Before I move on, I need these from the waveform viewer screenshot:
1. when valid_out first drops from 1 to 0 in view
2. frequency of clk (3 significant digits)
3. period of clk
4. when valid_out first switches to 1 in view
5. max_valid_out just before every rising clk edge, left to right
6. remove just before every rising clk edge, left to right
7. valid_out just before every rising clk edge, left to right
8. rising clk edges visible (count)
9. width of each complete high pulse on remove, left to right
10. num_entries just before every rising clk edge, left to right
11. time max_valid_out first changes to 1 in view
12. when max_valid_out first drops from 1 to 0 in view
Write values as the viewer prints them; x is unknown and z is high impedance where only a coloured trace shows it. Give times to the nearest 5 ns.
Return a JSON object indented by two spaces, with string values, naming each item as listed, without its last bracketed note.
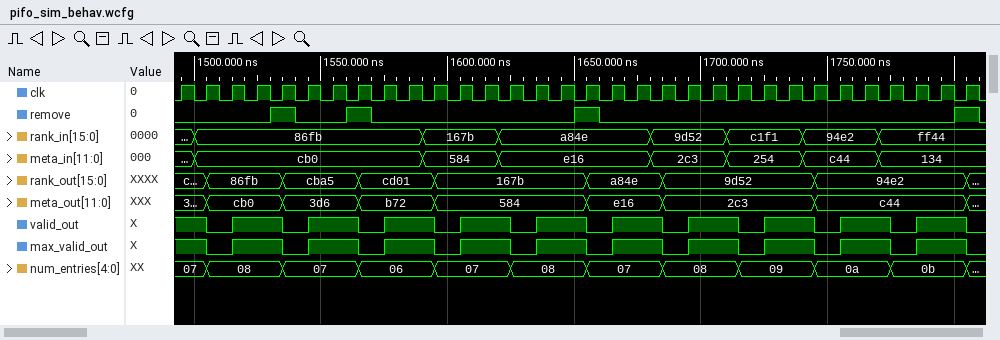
{
  "when valid_out first drops from 1 to 0 in view": "1505 ns",
  "frequency of clk": "100 MHz",
  "period of clk": "10 ns",
  "when valid_out first switches to 1 in view": "1515 ns",
  "max_valid_out just before every rising clk edge, left to right": "1 1 0 1 1 0 1 1 0 1 1 0 1 1 0 1 1 0 1 1 0 1 1 0 1 1 0 1 1 0 1 1",
  "remove just before every rising clk edge, left to right": "0 0 0 0 1 0 0 1 0 0 0 0 0 0 0 0 1 0 0 0 0 0 0 0 0 0 0 0 0 0 0 1",
  "valid_out just before every rising clk edge, left to right": "1 1 0 1 1 0 1 1 0 1 1 0 1 1 0 1 1 0 1 1 0 1 1 0 1 1 0 1 1 0 1 1",
  "rising clk edges visible": "32",
  "width of each complete high pulse on remove, left to right": "10 ns, 10 ns, 10 ns, 10 ns",
  "num_entries just before every rising clk edge, left to right": "07, 07, 08, 08, 08, 07, 07, 07, 06, 06, 06, 07, 07, 07, 08, 08, 08, 07, 07, 07, 08, 08, 08, 09, 09, 09, 0a, 0a, 0a, 0b, 0b, 0b",
  "time max_valid_out first changes to 1 in view": "1515 ns",
  "when max_valid_out first drops from 1 to 0 in view": "1505 ns"
}
